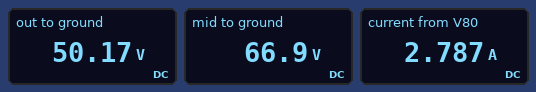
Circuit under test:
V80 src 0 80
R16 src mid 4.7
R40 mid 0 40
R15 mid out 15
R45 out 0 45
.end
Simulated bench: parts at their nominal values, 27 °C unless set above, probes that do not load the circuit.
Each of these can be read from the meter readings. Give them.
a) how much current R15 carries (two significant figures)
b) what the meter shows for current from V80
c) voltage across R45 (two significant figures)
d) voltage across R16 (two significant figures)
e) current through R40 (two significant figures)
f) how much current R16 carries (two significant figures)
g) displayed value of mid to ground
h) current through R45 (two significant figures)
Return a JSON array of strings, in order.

["1.1 A", "2.787 A", "50 V", "13 V", "1.7 A", "2.8 A", "66.9 V", "1.1 A"]
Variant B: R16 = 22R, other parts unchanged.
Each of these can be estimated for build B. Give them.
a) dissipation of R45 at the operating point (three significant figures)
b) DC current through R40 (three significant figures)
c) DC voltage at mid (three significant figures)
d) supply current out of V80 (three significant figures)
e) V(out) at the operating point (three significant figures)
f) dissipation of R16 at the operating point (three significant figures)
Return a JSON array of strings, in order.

["21.8 W", "1.04 A", "41.7 V", "1.74 A", "31.3 V", "66.5 W"]
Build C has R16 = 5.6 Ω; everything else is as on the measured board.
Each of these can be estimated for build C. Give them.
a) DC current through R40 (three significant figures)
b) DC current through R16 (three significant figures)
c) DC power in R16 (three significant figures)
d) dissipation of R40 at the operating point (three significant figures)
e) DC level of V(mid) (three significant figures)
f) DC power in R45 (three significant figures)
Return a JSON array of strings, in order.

["1.62 A", "2.70 A", "40.9 W", "105 W", "64.9 V", "52.6 W"]
